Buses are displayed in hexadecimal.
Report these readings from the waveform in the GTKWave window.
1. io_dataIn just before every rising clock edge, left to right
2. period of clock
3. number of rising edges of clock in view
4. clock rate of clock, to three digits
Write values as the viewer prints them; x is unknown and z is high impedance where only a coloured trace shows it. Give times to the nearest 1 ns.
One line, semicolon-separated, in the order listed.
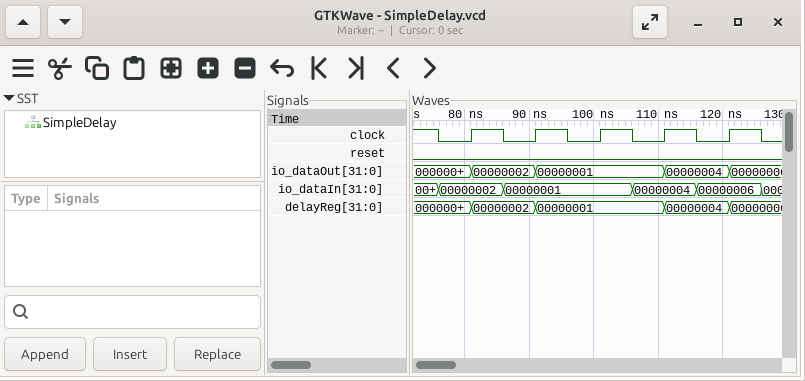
00000002, 00000001, 00000001, 00000004, 00000006; 10 ns; 5; 100 MHz
